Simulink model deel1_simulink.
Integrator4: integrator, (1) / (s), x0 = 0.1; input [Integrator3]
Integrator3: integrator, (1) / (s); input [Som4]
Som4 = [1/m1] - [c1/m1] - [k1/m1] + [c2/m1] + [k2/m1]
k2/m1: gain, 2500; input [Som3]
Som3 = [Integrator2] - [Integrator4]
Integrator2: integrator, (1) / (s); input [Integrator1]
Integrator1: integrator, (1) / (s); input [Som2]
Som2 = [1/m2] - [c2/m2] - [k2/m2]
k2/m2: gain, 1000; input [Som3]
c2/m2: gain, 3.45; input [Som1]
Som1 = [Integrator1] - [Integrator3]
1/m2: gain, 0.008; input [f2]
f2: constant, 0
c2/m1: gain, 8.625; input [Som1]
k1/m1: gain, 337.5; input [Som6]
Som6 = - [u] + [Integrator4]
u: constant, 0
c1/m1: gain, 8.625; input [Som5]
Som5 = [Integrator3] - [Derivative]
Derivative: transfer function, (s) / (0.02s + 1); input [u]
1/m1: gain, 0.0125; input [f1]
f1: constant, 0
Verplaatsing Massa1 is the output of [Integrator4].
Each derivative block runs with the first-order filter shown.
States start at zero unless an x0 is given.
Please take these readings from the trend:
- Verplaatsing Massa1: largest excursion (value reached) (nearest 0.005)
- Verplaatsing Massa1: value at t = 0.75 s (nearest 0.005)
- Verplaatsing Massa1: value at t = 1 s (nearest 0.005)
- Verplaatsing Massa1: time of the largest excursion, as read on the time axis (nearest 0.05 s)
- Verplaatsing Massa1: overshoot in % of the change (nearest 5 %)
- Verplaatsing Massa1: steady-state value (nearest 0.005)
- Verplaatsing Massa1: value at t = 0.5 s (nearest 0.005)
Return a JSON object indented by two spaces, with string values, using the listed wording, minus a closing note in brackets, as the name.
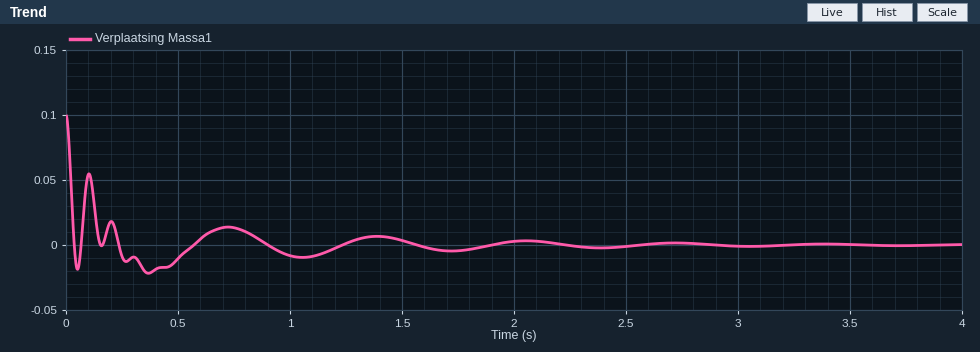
{
  "Verplaatsing Massa1: largest excursion (value reached)": "-0.020",
  "Verplaatsing Massa1: value at t = 0.75 s": "0.015",
  "Verplaatsing Massa1: value at t = 1 s": "-0.010",
  "Verplaatsing Massa1: time of the largest excursion, as read on the time axis": "0.35 s",
  "Verplaatsing Massa1: overshoot in % of the change": "20 %",
  "Verplaatsing Massa1: steady-state value": "0.000",
  "Verplaatsing Massa1: value at t = 0.5 s": "-0.010"
}
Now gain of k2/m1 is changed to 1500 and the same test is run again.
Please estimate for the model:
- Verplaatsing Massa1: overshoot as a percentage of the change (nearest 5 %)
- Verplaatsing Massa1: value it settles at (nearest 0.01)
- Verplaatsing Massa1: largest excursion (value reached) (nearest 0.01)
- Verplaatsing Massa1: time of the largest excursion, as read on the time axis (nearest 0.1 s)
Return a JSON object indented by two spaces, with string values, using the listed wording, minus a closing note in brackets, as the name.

{
  "Verplaatsing Massa1: overshoot as a percentage of the change": "30 %",
  "Verplaatsing Massa1: value it settles at": "0.00",
  "Verplaatsing Massa1: largest excursion (value reached)": "-0.03",
  "Verplaatsing Massa1: time of the largest excursion, as read on the time axis": "0.3 s"
}
